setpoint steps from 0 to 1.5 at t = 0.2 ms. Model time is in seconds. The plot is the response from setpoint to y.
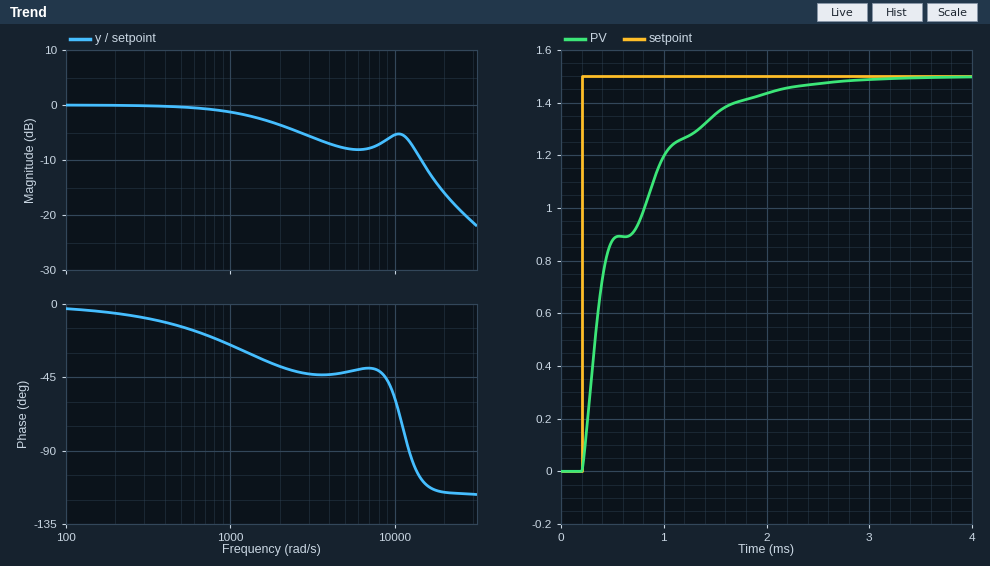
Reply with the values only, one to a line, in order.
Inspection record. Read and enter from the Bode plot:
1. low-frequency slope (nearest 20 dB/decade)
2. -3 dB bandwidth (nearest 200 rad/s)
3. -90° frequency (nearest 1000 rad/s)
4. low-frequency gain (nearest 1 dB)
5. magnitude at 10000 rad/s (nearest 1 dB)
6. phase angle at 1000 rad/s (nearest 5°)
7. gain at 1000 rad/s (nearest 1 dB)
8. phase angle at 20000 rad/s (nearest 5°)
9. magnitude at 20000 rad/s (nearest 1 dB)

0 dB/decade
1800 rad/s
12000 rad/s
0 dB
-5 dB
-25°
-1 dB
-115°
-16 dB
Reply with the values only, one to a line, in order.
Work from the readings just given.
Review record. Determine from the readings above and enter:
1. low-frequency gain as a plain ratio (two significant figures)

1.0
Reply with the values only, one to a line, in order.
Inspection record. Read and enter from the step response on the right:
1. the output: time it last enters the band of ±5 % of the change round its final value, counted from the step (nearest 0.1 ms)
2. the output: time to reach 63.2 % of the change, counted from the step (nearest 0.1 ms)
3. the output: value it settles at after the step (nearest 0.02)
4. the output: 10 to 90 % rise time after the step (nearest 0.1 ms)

1.7 ms
0.6 ms
1.50
1.2 ms
